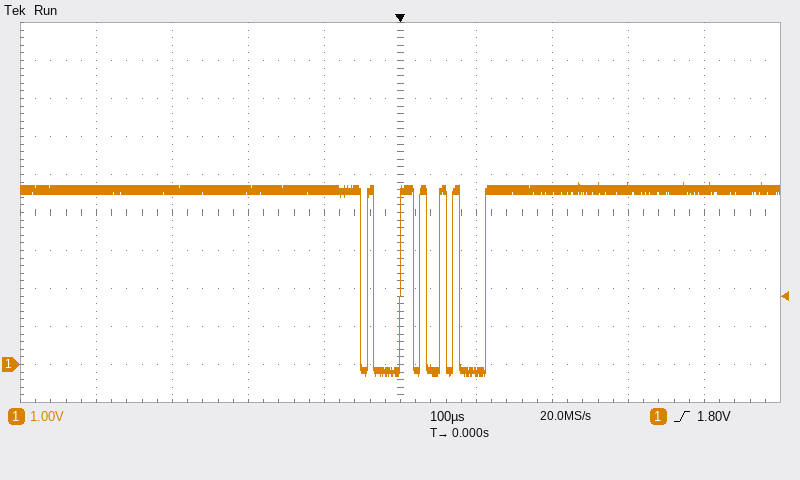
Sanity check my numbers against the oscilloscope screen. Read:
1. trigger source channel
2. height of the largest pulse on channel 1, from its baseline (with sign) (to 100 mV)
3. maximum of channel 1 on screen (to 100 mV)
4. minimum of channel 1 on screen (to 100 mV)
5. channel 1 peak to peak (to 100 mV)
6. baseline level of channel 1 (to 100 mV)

channel 1
-4.9 V
4.8 V
-300 mV
5.1 V
4.6 V
